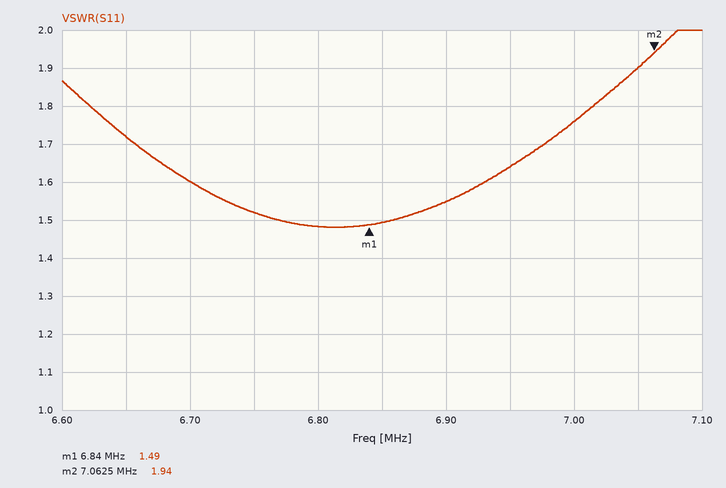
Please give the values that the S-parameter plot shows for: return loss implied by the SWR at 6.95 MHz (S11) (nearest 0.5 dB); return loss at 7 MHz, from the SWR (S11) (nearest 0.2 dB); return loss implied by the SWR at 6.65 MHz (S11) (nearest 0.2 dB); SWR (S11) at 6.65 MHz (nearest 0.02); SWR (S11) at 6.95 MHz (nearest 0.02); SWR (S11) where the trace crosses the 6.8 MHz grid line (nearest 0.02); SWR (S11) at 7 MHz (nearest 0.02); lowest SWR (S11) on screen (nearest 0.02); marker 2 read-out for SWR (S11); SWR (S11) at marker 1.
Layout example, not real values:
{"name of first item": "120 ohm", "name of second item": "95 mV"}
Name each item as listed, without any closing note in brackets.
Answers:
{"return loss implied by the SWR at 6.95 MHz (S11)": "12.5 dB", "return loss at 7 MHz, from the SWR (S11)": "11.2 dB", "return loss implied by the SWR at 6.65 MHz (S11)": "11.6 dB", "SWR (S11) at 6.65 MHz": "1.72", "SWR (S11) at 6.95 MHz": "1.64", "SWR (S11) where the trace crosses the 6.8 MHz grid line": "1.48", "SWR (S11) at 7 MHz": "1.76", "lowest SWR (S11) on screen": "1.48", "marker 2 read-out for SWR": "1.94", "SWR (S11) at marker 1": "1.49"}
